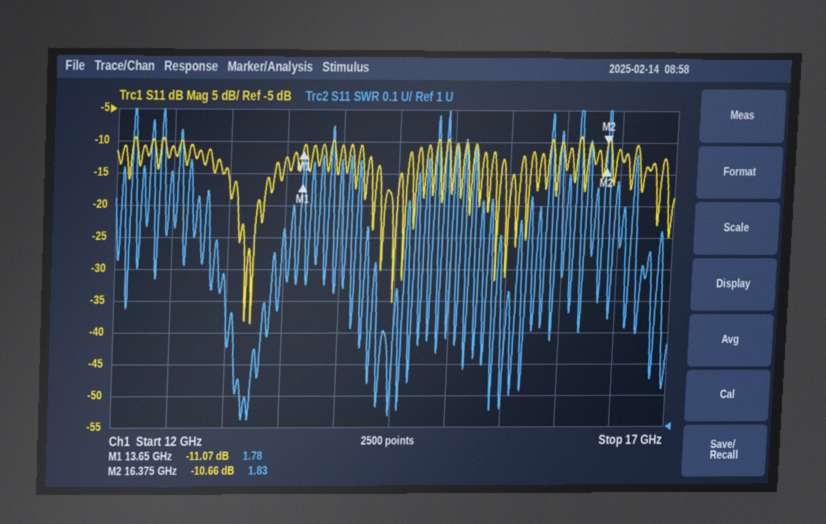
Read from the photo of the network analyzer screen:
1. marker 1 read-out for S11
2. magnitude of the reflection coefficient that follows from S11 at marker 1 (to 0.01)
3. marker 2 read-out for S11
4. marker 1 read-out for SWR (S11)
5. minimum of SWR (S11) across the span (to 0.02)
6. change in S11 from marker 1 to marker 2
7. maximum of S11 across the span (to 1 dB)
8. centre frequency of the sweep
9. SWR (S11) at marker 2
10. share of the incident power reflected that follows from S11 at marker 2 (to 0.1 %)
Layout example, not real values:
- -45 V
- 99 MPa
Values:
- -11.07 dB
- 0.28
- -10.66 dB
- 1.78
- 1.02
- 0.41 dB
- -9 dB
- 14.5 GHz
- 1.83
- 8.6 %
